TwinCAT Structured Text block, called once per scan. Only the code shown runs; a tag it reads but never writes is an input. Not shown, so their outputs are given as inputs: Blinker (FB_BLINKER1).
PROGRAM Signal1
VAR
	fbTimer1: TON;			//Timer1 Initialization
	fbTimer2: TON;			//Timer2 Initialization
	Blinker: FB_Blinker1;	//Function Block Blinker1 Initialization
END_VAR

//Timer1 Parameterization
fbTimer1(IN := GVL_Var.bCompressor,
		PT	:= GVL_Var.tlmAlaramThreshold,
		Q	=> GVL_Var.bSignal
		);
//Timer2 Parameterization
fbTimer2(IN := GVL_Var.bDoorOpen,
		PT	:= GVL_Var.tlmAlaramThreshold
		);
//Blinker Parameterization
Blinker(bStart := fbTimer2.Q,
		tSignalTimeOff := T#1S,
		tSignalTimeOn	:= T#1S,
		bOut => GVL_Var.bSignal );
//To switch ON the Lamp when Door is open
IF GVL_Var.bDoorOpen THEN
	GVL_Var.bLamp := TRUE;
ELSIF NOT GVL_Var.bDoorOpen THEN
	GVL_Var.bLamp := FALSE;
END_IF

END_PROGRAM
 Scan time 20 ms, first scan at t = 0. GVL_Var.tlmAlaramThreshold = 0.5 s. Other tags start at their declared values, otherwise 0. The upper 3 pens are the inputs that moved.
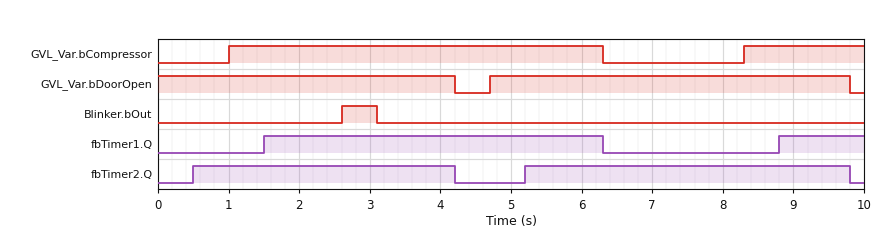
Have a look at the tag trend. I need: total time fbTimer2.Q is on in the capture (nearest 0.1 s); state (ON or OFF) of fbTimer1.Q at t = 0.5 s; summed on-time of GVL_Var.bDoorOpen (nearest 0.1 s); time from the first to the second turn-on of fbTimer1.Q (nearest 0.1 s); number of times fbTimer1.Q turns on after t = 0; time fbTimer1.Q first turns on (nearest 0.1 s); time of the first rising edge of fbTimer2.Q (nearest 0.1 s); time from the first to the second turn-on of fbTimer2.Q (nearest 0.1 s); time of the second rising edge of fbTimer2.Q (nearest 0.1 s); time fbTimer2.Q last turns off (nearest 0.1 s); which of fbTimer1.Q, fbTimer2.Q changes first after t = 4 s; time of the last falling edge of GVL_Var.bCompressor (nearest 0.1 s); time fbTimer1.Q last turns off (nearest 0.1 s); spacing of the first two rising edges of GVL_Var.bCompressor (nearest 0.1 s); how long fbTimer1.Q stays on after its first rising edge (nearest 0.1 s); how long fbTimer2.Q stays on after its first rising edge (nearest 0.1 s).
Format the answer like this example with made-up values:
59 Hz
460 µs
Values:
8.3 s
OFF
9.3 s
7.3 s
2
1.5 s
0.5 s
4.7 s
5.2 s
9.8 s
fbTimer2.Q
6.3 s
6.3 s
7.3 s
4.8 s
3.7 s
